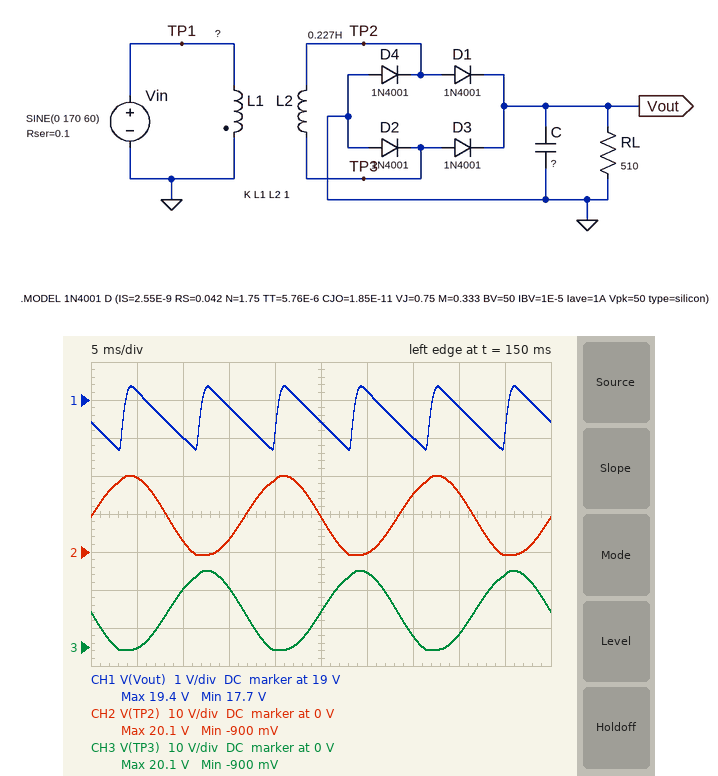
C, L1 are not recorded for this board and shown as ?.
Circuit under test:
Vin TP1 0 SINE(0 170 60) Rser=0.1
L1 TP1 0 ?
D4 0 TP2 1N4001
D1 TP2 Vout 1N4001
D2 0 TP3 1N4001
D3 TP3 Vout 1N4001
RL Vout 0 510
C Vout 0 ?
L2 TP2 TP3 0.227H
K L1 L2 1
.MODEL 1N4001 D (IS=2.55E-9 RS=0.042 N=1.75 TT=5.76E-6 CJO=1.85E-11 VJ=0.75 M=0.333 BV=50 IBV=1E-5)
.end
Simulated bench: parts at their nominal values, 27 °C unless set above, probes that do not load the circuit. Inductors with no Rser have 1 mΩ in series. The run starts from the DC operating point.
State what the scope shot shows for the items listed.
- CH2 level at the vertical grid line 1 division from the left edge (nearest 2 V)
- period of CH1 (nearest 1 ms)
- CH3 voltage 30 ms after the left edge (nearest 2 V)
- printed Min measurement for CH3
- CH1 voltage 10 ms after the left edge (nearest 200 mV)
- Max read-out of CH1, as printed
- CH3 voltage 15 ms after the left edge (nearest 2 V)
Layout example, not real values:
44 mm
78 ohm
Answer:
20 V
8 ms
20 V
-900 mV
18.0 V
19.4 V
16 V
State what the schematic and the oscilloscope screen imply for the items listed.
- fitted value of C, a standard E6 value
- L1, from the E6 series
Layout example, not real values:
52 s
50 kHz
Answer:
150 µF
15 H
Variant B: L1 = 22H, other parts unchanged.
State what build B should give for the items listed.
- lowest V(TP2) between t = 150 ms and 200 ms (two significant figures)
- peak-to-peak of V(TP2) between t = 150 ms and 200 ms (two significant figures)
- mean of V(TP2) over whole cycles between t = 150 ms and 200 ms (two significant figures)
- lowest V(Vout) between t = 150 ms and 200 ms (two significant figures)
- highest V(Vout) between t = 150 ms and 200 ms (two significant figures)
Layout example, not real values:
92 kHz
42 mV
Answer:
-860 mV
17 V
7.5 V
14 V
16 V
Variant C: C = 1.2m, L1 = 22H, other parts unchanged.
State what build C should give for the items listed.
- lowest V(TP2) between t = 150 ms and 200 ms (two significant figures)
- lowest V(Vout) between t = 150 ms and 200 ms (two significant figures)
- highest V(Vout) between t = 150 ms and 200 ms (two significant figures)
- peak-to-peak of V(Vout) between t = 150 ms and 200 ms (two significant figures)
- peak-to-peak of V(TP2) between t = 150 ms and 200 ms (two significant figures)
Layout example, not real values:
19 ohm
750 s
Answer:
-880 mV
15 V
16 V
180 mV
17 V
